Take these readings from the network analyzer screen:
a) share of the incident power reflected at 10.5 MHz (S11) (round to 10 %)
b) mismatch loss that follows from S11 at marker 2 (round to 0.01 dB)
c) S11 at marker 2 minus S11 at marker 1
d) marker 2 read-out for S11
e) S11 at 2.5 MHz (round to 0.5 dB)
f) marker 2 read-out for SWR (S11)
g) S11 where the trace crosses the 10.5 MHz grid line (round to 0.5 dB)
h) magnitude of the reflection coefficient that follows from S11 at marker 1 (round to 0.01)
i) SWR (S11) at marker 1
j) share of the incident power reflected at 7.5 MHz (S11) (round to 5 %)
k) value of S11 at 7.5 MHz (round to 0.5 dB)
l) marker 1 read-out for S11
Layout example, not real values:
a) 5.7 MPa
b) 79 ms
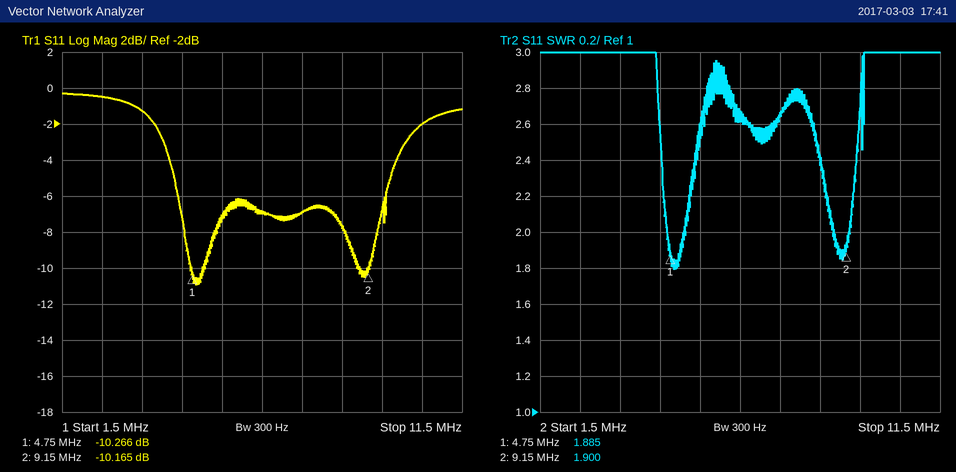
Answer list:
a) 60 %
b) 0.44 dB
c) 0.101 dB
d) -10.165 dB
e) -0.5 dB
f) 1.900
g) -2.0 dB
h) 0.31
i) 1.885
j) 20 %
k) -7.0 dB
l) -10.266 dB
